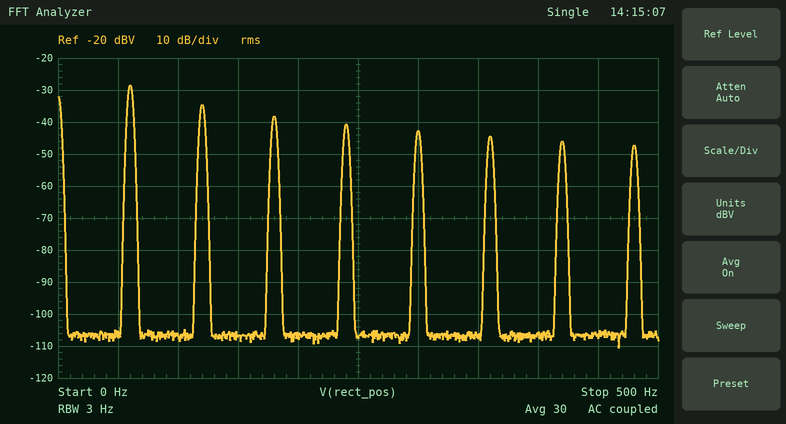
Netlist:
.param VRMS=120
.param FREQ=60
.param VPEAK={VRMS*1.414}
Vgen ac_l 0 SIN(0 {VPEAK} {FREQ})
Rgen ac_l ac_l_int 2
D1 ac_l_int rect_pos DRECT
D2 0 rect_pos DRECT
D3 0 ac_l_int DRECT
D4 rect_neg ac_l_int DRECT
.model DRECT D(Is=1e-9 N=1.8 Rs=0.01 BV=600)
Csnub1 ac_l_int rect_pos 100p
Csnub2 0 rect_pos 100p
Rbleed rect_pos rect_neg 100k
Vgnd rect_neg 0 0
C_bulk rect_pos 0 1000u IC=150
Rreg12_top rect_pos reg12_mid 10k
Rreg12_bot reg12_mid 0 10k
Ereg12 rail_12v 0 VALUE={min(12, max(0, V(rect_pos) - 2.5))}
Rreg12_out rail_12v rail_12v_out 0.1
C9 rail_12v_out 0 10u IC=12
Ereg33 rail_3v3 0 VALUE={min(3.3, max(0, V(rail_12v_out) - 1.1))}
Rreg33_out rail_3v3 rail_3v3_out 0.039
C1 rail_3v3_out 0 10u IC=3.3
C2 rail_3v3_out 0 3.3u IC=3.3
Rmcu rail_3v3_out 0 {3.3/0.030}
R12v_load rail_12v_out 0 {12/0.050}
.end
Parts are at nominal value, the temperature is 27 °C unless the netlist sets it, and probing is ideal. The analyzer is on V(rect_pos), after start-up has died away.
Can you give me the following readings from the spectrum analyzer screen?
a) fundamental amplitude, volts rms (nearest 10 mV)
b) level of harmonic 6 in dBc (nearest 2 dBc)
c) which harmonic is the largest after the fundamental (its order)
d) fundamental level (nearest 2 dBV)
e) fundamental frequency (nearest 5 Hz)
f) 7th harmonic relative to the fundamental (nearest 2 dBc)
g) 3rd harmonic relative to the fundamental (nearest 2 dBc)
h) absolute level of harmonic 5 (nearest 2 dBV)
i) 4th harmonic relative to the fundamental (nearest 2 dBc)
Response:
40 mV
-16 dBc
2
-28 dBV
60 Hz
-18 dBc
-10 dBc
-42 dBV
-12 dBc
